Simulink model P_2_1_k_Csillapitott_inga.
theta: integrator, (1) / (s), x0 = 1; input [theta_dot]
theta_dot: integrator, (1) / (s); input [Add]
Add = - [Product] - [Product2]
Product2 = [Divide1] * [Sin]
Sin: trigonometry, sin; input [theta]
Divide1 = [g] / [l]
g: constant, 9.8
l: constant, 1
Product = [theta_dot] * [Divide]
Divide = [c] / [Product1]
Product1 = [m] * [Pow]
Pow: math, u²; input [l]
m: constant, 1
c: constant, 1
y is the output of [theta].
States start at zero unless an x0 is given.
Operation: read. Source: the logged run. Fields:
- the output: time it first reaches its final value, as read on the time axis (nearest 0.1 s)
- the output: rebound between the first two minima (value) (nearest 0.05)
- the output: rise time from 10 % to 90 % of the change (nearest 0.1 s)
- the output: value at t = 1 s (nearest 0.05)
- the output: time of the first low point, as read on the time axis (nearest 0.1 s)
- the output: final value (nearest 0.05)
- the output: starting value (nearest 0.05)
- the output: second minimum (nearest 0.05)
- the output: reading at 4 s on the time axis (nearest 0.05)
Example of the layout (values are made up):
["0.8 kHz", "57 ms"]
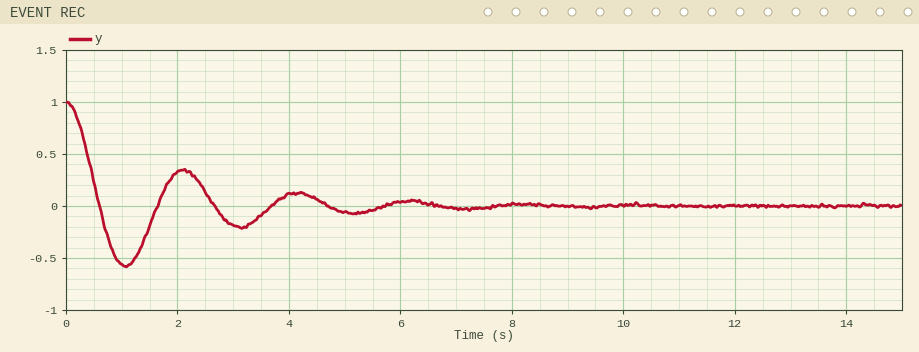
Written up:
["0.6 s", "0.35", "0.4 s", "-0.55", "1.1 s", "0.00", "1.00", "-0.20", "0.10"]
